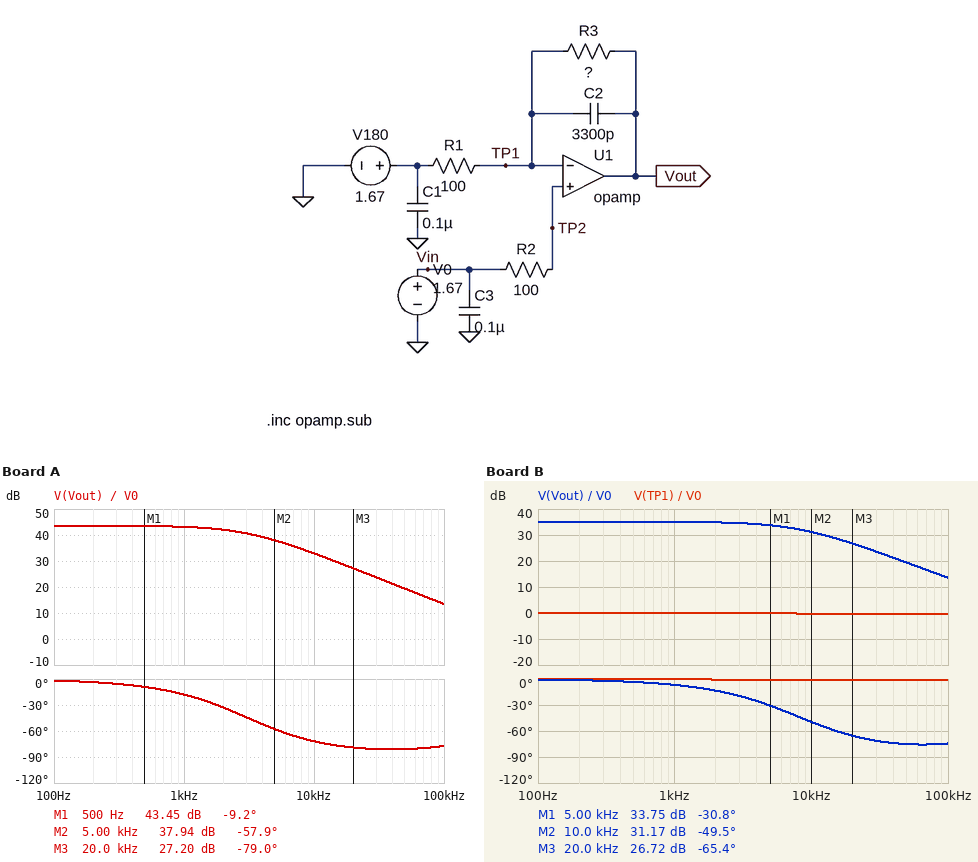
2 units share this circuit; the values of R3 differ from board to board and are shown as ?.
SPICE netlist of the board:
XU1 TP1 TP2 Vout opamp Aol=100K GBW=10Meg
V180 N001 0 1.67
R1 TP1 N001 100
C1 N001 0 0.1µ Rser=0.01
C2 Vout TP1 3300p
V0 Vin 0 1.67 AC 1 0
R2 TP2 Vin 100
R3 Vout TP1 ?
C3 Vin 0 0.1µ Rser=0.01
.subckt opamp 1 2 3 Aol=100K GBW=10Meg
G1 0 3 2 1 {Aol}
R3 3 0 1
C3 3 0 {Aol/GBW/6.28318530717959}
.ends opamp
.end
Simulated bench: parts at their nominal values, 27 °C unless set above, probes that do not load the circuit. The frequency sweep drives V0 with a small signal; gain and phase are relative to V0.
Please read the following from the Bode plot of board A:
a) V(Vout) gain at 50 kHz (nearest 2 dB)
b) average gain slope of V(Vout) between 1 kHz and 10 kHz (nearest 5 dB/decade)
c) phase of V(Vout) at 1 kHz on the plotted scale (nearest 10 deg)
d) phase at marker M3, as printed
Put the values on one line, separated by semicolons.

20 dB; -10 dB/decade; -20 deg; -79.0 deg
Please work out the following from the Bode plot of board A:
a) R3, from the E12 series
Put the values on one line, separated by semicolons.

15 kΩ
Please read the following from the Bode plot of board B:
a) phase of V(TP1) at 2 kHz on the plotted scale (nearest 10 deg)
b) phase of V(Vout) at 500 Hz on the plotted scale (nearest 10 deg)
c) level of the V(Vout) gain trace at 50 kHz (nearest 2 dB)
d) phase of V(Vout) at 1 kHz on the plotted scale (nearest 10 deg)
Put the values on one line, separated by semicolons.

0 deg; 0 deg; 20 dB; -10 deg
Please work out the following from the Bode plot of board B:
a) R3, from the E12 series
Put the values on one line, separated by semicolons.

5.6 kΩ
